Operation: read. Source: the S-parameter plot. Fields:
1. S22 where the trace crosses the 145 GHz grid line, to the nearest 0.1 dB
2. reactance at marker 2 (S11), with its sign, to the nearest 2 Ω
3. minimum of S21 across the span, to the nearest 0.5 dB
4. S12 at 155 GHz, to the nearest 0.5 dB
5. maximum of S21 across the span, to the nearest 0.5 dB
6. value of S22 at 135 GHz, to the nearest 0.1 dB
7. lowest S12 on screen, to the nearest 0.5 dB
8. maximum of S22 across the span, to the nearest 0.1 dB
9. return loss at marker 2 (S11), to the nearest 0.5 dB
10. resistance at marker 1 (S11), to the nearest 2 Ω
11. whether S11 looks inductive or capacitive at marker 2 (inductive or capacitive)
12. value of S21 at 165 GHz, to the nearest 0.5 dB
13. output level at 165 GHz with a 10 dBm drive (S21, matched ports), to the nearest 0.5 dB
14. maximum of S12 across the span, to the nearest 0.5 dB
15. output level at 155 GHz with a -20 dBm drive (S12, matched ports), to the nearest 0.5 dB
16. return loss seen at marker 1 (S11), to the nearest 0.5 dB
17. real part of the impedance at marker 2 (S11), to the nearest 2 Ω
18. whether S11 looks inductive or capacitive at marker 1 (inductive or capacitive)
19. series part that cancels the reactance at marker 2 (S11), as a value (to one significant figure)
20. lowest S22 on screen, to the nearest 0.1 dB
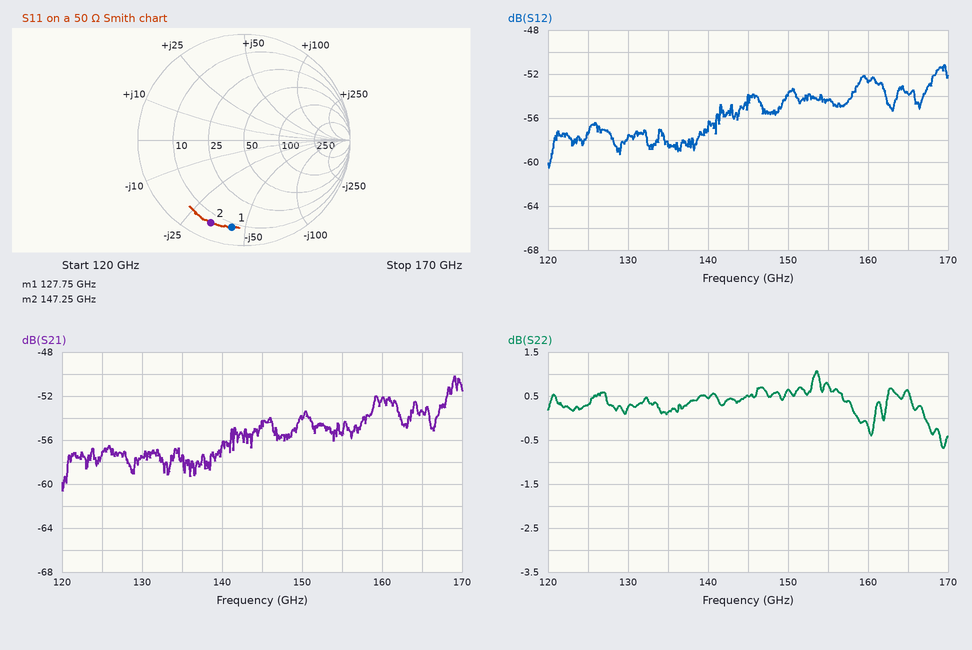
0.5 dB
-34 Ω
-60.5 dB
-54.5 dB
-50.0 dB
0.1 dB
-60.5 dB
1.1 dB
1.5 dB
8 Ω
capacitive
-53.5 dB
-43.5 dBm
-51.0 dB
-74.5 dBm
1.5 dB
6 Ω
capacitive
40 pH
-0.7 dB
